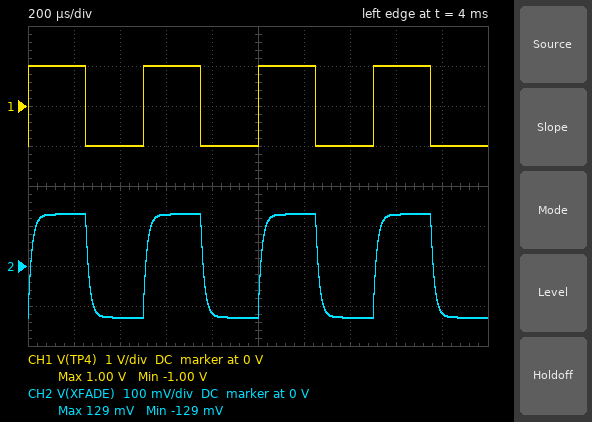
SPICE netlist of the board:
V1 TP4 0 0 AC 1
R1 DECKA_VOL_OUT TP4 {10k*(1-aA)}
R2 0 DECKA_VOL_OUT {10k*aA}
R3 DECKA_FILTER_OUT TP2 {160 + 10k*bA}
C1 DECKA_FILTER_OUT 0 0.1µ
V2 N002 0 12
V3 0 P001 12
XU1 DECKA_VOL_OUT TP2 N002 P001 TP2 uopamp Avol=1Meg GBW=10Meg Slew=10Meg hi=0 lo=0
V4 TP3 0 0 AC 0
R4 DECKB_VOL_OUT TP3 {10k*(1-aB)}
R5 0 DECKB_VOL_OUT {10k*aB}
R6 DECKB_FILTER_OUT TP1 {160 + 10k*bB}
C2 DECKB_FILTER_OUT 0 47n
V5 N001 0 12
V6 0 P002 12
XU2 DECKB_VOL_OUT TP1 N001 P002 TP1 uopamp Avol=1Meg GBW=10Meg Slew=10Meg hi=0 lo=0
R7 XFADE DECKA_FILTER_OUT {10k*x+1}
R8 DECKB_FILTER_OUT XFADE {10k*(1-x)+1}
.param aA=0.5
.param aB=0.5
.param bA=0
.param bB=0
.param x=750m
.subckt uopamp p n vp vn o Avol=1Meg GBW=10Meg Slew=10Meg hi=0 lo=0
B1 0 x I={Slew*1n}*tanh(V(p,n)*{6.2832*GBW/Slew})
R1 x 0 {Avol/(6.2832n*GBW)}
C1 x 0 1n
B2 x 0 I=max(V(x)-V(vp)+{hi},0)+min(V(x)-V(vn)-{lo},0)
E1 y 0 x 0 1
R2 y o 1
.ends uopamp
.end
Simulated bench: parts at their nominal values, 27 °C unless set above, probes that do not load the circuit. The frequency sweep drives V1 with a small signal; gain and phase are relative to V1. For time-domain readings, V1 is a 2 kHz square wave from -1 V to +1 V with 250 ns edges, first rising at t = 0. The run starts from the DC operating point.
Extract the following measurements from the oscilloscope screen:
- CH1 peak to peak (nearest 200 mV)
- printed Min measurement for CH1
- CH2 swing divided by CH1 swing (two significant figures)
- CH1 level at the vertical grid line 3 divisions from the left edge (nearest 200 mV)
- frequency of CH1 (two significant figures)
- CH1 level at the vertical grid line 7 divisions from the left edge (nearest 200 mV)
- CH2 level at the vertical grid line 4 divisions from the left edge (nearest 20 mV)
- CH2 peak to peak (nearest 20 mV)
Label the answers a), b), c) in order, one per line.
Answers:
a) 2.0 V
b) -1.00 V
c) 0.13
d) 1.0 V
e) 2.0 kHz
f) -1.0 V
g) -120 mV
h) 260 mV
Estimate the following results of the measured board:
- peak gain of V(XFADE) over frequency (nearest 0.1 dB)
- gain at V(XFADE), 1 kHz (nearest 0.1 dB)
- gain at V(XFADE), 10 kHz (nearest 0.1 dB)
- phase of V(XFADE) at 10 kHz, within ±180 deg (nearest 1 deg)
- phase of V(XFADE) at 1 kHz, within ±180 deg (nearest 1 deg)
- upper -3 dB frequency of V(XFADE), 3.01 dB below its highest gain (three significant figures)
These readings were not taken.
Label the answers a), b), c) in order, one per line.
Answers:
a) -17.8 dB
b) -17.8 dB
c) -20.8 dB
d) -46 deg
e) -6 deg
f) 9.94 kHz
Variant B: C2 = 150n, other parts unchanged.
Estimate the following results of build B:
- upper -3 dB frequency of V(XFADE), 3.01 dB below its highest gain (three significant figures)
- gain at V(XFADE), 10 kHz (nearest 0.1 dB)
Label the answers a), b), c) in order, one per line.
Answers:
a) 9.49 kHz
b) -21.0 dB
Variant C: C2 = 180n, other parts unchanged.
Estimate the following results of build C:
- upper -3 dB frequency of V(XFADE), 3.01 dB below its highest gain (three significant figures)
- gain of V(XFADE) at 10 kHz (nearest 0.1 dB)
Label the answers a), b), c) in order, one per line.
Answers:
a) 9.42 kHz
b) -21.1 dB
